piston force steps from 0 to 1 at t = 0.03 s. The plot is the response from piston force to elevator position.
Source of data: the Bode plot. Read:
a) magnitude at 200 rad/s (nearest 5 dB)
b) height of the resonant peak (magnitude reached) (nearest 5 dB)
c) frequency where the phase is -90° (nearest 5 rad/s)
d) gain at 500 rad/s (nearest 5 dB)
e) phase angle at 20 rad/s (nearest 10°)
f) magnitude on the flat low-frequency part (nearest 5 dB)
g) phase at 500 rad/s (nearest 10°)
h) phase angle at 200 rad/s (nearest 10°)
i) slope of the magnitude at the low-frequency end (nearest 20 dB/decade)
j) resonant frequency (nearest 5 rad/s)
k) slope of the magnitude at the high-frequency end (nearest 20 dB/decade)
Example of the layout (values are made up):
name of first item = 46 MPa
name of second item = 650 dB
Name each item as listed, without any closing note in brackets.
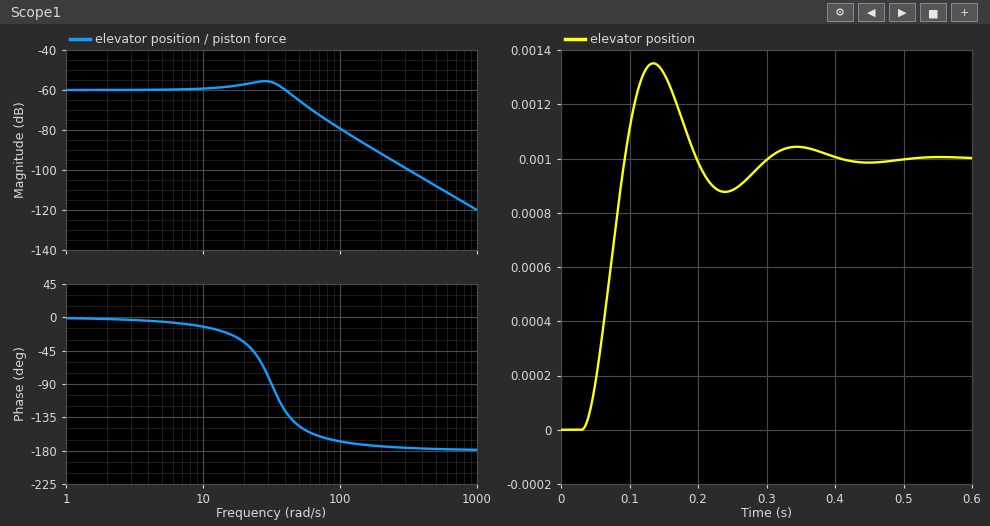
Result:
magnitude at 200 rad/s = -90 dB
height of the resonant peak (magnitude reached) = -55 dB
frequency where the phase is -90° = 30 rad/s
gain at 500 rad/s = -110 dB
phase angle at 20 rad/s = -30°
magnitude on the flat low-frequency part = -60 dB
phase at 500 rad/s = -180°
phase angle at 200 rad/s = -170°
slope of the magnitude at the low-frequency end = 0 dB/decade
resonant frequency = 30 rad/s
slope of the magnitude at the high-frequency end = -40 dB/decade
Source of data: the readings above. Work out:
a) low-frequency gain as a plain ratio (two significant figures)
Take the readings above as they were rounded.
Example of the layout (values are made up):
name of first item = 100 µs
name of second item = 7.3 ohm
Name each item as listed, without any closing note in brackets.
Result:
low-frequency gain as a plain ratio = 0.0010
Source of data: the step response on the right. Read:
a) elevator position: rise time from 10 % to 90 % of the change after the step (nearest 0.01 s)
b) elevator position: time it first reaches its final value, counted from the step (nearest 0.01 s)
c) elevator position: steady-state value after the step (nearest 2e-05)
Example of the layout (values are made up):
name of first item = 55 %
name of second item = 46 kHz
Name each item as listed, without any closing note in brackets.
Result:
elevator position: rise time from 10 % to 90 % of the change after the step = 0.04 s
elevator position: time it first reaches its final value, counted from the step = 0.06 s
elevator position: steady-state value after the step = 0.00100
